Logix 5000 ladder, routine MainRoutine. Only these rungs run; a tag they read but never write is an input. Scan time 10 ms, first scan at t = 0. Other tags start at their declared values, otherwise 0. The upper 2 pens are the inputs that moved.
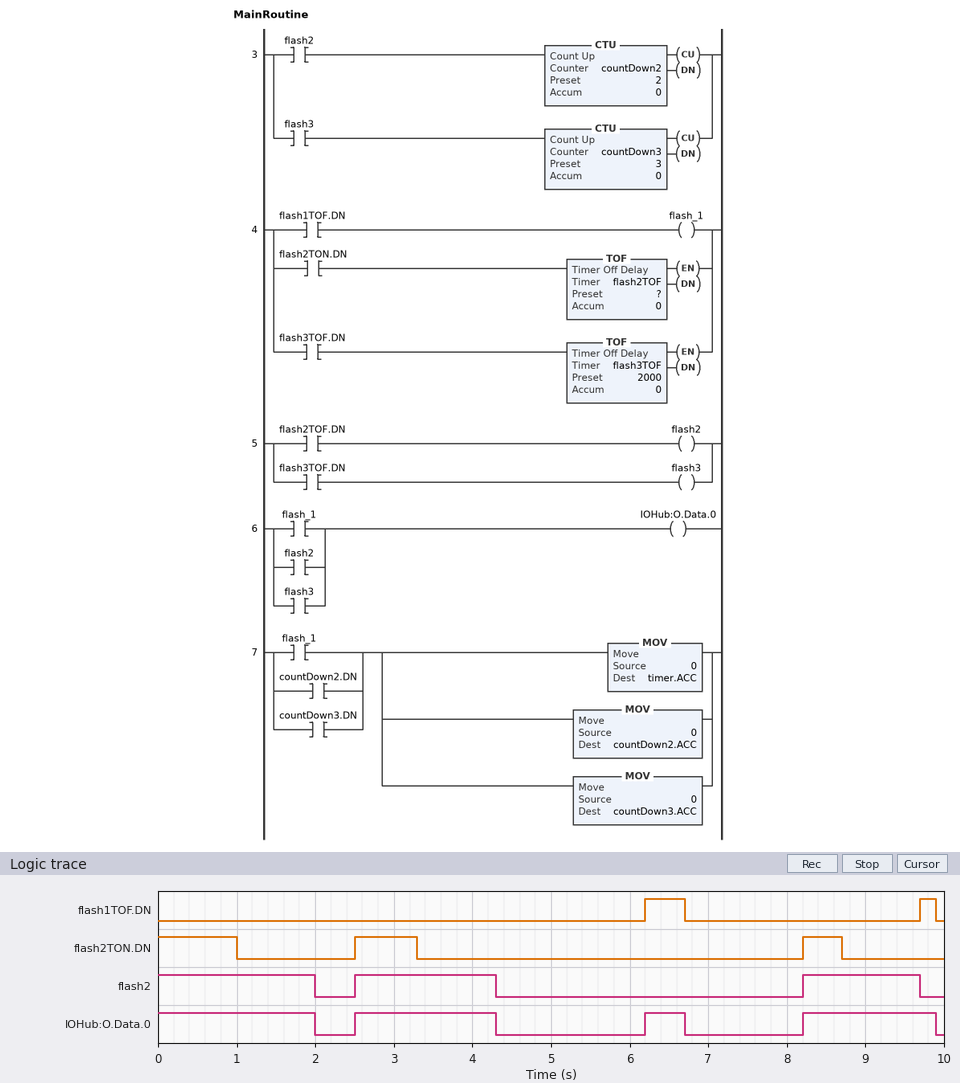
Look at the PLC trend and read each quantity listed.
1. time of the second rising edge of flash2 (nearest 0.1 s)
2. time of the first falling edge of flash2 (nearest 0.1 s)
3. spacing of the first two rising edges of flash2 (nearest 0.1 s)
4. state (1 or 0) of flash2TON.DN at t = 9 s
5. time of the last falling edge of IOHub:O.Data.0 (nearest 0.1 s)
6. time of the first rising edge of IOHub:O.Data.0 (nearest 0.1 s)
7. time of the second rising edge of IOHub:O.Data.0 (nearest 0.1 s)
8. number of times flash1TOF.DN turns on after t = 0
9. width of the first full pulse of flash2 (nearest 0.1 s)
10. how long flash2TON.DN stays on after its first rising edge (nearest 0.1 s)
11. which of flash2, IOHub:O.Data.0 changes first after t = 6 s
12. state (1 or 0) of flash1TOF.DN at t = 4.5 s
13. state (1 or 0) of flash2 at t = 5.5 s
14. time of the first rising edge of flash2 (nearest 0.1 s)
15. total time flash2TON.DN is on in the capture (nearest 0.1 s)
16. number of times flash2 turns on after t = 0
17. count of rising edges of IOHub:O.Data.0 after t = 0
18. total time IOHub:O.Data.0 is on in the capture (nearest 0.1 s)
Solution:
8.2 s
2.0 s
5.7 s
0
9.9 s
2.5 s
6.2 s
2
1.8 s
0.8 s
IOHub:O.Data.0
0
0
2.5 s
2.3 s
2
3
6.0 s
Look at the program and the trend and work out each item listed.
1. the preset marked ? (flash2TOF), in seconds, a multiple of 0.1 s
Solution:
1.0 s
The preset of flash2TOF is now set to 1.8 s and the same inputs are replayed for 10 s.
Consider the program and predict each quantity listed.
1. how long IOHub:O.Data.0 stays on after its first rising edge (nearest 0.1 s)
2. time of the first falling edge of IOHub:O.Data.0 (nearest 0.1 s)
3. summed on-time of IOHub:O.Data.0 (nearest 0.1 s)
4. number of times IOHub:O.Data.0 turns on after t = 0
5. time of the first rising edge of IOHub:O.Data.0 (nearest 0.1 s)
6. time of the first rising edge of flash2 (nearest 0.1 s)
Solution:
0.5 s
5.1 s
7.4 s
2
6.2 s
8.2 s
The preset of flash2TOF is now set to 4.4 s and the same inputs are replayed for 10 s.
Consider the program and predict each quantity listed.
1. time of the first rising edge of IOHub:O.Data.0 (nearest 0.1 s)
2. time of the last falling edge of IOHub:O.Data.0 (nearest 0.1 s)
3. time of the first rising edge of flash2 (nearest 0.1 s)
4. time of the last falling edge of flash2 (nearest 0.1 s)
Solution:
8.2 s
7.7 s
8.2 s
7.7 s
